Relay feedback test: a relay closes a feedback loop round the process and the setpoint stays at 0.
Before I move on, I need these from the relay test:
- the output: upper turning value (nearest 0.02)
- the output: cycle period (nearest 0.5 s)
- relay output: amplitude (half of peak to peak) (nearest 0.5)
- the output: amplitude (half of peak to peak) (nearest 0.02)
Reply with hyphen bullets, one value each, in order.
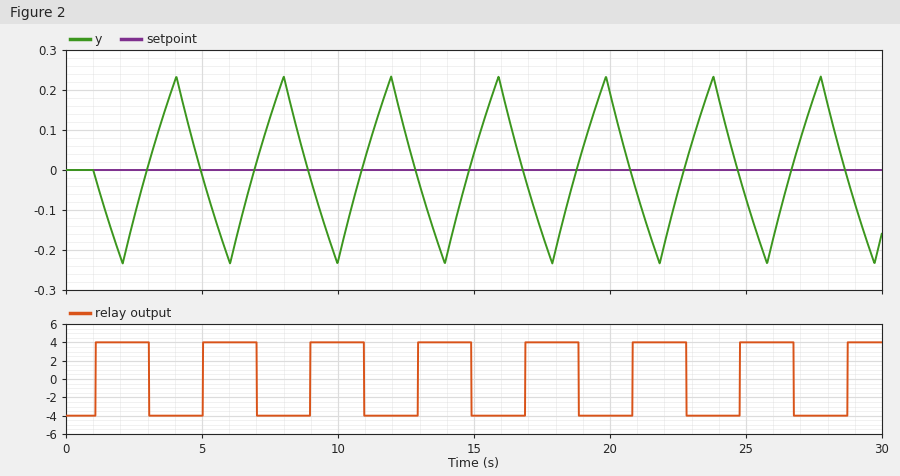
- 0.24
- 4.0 s
- 4.0
- 0.24
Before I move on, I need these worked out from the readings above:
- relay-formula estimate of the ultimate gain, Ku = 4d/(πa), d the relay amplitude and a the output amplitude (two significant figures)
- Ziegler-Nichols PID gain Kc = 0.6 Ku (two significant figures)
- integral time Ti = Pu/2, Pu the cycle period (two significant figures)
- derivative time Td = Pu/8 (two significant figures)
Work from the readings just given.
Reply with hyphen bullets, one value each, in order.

- 21
- 13
- 2.0 s
- 0.50 s
